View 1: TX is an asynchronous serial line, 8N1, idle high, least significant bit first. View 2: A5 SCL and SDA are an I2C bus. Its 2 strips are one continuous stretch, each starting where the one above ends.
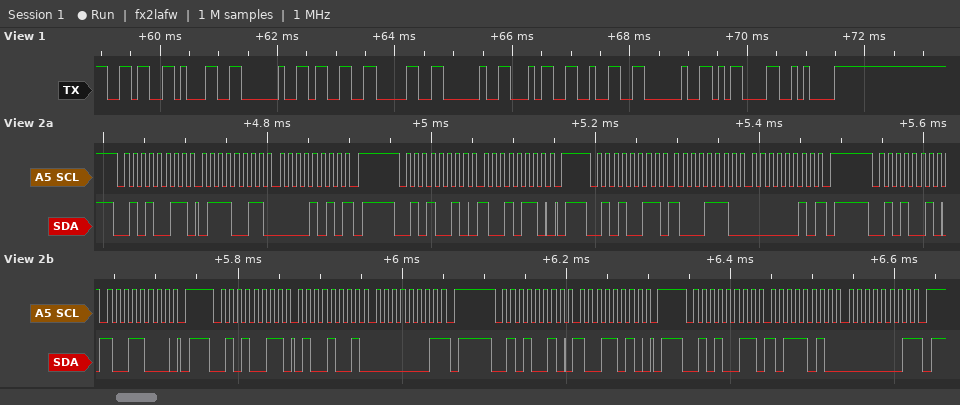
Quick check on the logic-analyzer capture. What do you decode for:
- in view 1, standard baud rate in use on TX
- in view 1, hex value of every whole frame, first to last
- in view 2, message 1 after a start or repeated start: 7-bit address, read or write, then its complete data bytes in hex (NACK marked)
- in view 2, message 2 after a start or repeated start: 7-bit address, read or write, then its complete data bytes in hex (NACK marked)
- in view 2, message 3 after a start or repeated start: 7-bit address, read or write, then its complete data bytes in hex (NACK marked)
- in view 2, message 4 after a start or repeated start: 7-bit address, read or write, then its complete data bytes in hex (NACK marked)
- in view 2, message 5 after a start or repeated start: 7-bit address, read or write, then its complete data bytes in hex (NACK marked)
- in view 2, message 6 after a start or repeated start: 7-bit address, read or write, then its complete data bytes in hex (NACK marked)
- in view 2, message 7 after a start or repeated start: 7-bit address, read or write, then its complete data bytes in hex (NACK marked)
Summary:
9600 baud
36 31 20 33 30 20 34 32 20 0D 0A
0x29 read: 73 0A NACK
0x29 write: 96
0x29 read: 8E 02 NACK
0x29 write: 98
0x29 read: 49 01 NACK
0x29 write: 9A
0x29 read: BA 01 NACK
